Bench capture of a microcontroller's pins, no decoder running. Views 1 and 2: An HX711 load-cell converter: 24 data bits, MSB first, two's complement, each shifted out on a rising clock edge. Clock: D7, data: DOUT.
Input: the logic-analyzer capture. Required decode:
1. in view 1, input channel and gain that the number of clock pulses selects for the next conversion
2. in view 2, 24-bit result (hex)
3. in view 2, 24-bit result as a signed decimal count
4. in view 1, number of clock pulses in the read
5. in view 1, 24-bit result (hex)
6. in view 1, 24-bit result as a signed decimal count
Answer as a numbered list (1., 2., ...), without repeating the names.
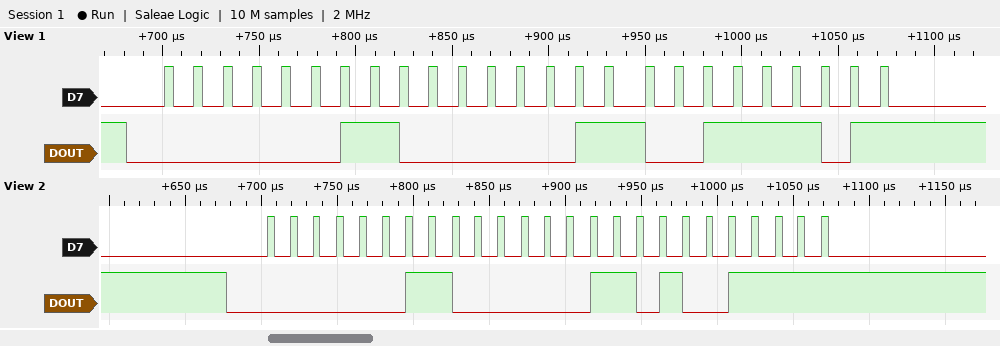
1. channel A, gain 128
2. 0x03034F
3. 197455
4. 25
5. 0x03033D
6. 197437
